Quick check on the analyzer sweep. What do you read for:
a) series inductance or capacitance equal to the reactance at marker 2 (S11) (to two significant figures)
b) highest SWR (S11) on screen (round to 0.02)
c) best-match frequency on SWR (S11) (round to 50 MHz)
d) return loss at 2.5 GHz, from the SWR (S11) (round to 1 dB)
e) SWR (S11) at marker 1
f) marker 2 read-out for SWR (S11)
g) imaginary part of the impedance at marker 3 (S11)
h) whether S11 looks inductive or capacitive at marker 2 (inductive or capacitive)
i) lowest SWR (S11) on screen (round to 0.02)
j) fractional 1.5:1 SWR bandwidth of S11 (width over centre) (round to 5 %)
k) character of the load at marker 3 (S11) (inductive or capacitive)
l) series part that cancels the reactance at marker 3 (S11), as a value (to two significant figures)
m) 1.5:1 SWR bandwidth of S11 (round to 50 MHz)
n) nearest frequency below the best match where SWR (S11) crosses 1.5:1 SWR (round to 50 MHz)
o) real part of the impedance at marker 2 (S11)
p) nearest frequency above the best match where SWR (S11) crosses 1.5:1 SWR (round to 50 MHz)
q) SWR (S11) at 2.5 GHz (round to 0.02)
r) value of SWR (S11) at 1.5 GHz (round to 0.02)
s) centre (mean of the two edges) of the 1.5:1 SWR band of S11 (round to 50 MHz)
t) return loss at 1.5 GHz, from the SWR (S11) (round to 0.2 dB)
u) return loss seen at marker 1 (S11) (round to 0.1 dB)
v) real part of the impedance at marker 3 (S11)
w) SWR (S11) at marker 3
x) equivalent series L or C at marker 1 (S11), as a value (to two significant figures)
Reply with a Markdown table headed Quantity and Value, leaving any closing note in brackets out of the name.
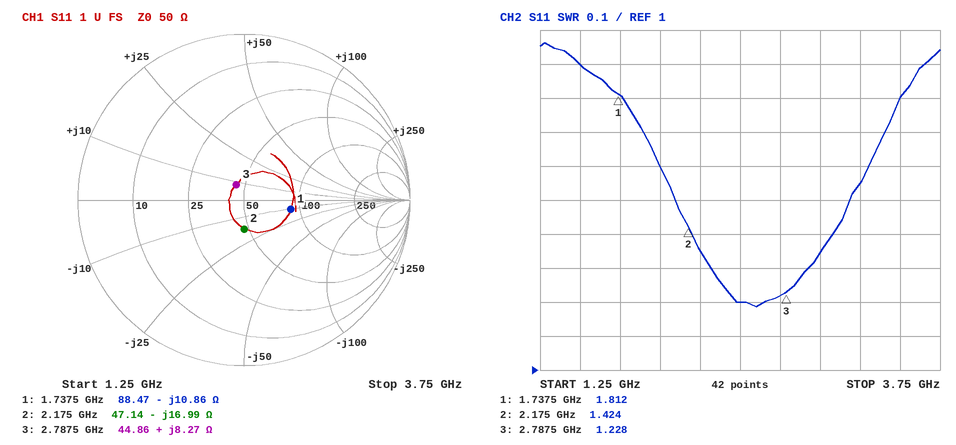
| Quantity | Value |
|---|---|
| series inductance or capacitance equal to the reactance at marker 2 (S11) | 4.3 pF |
| highest SWR (S11) on screen | 1.96 |
| best-match frequency on SWR (S11) | 2.60 GHz |
| return loss at 2.5 GHz, from the SWR (S11) | 21 dB |
| SWR (S11) at marker 1 | 1.812 |
| marker 2 read-out for SWR | 1.424 |
| imaginary part of the impedance at marker 3 | +8.27 Ω |
| whether S11 looks inductive or capacitive at marker 2 | capacitive |
| lowest SWR (S11) on screen | 1.18 |
| fractional 1.5:1 SWR bandwidth of S11 (width over centre) | 40 % |
| character of the load at marker 3 (S11) | inductive |
| series part that cancels the reactance at marker 3 (S11), as a value | 6.9 pF |
| 1.5:1 SWR bandwidth of S11 | 1.10 GHz |
| nearest frequency below the best match where SWR (S11) crosses 1.5:1 SWR | 2.10 GHz |
| real part of the impedance at marker 2 | 47.14 Ω |
| nearest frequency above the best match where SWR (S11) crosses 1.5:1 SWR | 3.20 GHz |
| SWR (S11) at 2.5 GHz | 1.20 |
| value of SWR (S11) at 1.5 GHz | 1.90 |
| centre (mean of the two edges) of the 1.5:1 SWR band of S11 | 2.65 GHz |
| return loss at 1.5 GHz, from the SWR (S11) | 10.2 dB |
| return loss seen at marker 1 (S11) | 10.8 dB |
| real part of the impedance at marker 3 | 44.86 Ω |
| SWR (S11) at marker 3 | 1.228 |
| equivalent series L or C at marker 1 (S11), as a value | 8.4 pF |
